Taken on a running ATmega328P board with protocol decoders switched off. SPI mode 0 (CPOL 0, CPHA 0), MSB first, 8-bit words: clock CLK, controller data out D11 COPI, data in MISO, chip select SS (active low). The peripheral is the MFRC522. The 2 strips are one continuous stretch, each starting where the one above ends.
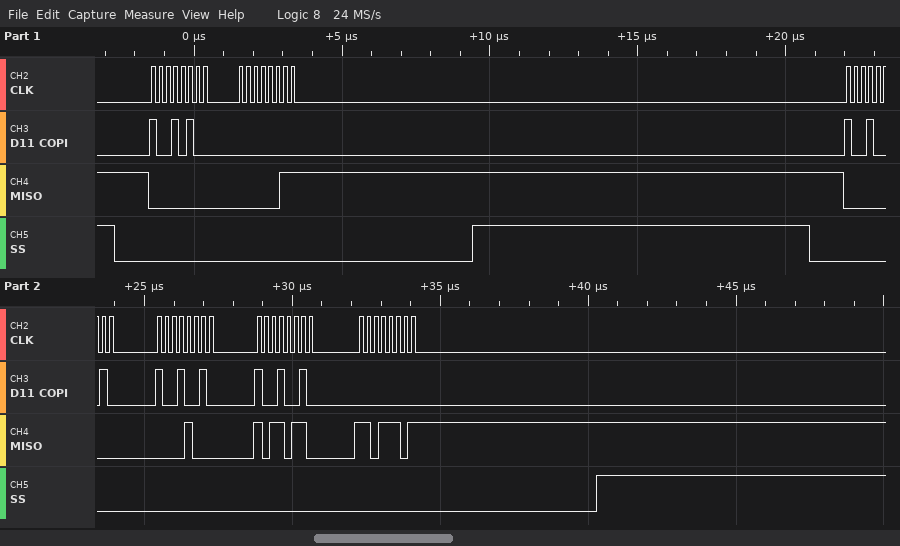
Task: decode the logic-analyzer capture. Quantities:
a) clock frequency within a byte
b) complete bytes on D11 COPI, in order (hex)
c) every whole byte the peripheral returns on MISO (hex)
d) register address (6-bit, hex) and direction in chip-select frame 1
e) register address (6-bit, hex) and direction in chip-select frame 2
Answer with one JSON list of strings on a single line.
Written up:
["4 MHz", "0x94 0x00 0x92 0x92 0x92 0x00", "0x00 0x03 0x00 0x08 0xB6 0xDD", "0x0A read", "0x09 read"]
